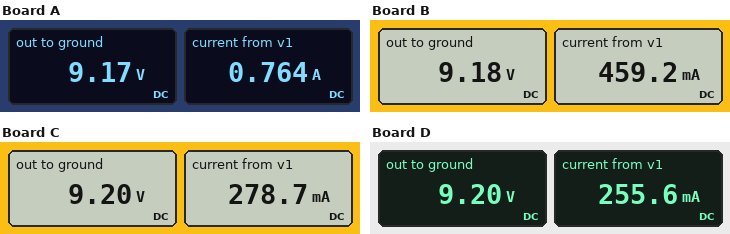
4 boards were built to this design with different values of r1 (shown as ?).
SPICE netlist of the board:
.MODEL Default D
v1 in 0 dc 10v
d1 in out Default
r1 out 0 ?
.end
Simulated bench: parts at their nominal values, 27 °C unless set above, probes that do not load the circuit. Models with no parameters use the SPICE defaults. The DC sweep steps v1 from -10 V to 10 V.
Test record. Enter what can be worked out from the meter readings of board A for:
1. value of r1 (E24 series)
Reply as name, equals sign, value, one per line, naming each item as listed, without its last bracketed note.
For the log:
value of r1 = 12 Ω
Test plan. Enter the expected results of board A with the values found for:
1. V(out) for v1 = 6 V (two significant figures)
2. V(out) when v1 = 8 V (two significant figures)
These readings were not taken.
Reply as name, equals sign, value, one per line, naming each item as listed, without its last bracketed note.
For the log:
V(out) for v1 = 6 V = 5.2 V
V(out) when v1 = 8 V = 7.2 V
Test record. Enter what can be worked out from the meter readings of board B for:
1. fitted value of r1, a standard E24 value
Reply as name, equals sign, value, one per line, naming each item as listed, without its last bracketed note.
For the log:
fitted value of r1, a standard E24 value = 20 Ω
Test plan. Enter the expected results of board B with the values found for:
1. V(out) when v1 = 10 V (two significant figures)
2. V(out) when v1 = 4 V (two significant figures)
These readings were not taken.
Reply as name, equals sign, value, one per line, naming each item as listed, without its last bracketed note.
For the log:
V(out) when v1 = 10 V = 9.2 V
V(out) when v1 = 4 V = 3.2 V
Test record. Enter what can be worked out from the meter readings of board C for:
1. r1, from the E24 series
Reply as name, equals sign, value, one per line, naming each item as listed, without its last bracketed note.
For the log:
r1, from the E24 series = 33 Ω
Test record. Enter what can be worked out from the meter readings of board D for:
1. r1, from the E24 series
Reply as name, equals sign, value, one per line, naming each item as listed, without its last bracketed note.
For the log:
r1, from the E24 series = 36 Ω
